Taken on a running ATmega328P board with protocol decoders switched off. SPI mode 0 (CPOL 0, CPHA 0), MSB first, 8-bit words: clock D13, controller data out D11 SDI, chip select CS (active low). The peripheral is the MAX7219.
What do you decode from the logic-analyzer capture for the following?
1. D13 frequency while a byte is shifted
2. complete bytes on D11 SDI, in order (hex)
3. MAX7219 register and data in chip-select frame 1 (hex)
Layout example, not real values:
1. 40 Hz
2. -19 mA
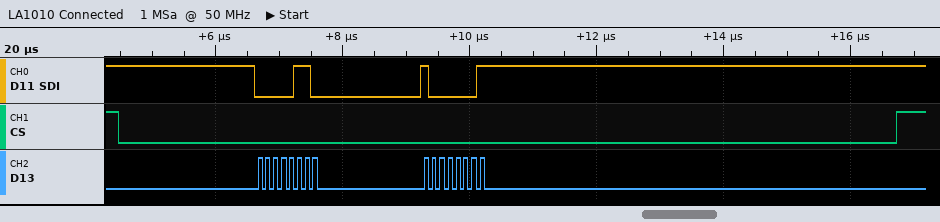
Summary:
1. 8 MHz
2. 06 81
3. register 0x6, data 0x81
